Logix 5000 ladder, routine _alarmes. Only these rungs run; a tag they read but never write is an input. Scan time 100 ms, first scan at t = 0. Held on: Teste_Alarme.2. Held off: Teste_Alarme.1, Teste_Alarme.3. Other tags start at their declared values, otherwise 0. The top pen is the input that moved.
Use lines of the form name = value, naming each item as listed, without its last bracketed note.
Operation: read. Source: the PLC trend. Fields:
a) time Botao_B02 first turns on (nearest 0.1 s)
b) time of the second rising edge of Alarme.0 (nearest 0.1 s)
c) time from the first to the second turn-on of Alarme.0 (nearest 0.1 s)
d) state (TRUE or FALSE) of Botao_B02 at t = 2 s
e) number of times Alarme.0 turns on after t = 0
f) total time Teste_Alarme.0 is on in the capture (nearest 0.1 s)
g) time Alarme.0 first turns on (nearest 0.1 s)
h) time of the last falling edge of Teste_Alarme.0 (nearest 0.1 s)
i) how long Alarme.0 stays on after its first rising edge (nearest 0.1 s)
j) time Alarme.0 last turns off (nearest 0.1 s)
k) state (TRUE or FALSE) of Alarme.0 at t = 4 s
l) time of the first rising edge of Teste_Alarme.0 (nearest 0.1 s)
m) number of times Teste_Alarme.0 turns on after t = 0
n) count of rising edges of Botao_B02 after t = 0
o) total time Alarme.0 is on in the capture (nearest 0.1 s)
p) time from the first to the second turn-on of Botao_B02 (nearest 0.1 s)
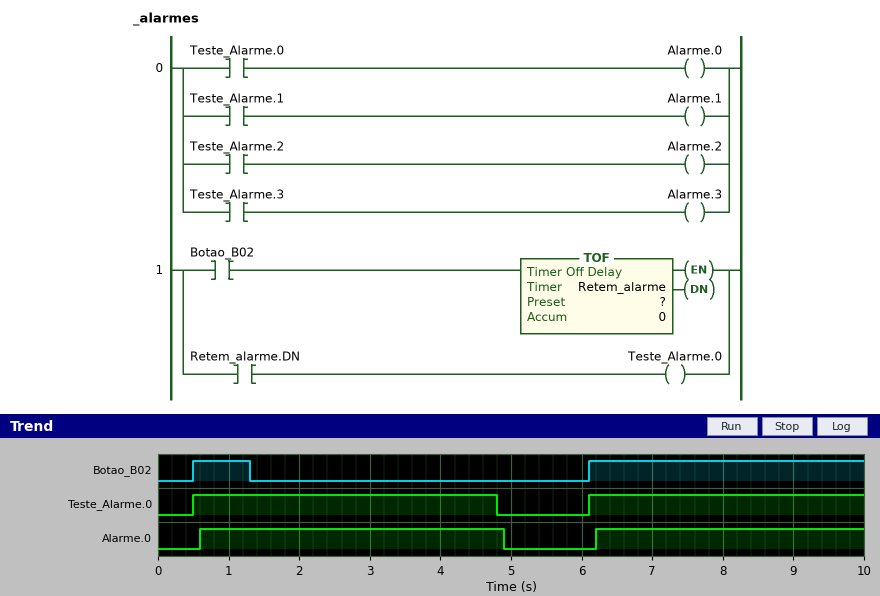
time Botao_B02 first turns on = 0.5 s
time of the second rising edge of Alarme.0 = 6.2 s
time from the first to the second turn-on of Alarme.0 = 5.6 s
state (TRUE or FALSE) of Botao_B02 at t = 2 s = FALSE
number of times Alarme.0 turns on after t = 0 = 2
total time Teste_Alarme.0 is on in the capture = 8.2 s
time Alarme.0 first turns on = 0.6 s
time of the last falling edge of Teste_Alarme.0 = 4.8 s
how long Alarme.0 stays on after its first rising edge = 4.3 s
time Alarme.0 last turns off = 4.9 s
state (TRUE or FALSE) of Alarme.0 at t = 4 s = TRUE
time of the first rising edge of Teste_Alarme.0 = 0.5 s
number of times Teste_Alarme.0 turns on after t = 0 = 2
count of rising edges of Botao_B02 after t = 0 = 2
total time Alarme.0 is on in the capture = 8.1 s
time from the first to the second turn-on of Botao_B02 = 5.6 s
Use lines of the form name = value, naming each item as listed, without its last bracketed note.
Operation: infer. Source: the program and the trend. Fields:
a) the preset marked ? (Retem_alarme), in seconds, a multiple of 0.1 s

the preset marked ? (Retem_alarme), in seconds, a multiple of 0.1 s = 3.5 s
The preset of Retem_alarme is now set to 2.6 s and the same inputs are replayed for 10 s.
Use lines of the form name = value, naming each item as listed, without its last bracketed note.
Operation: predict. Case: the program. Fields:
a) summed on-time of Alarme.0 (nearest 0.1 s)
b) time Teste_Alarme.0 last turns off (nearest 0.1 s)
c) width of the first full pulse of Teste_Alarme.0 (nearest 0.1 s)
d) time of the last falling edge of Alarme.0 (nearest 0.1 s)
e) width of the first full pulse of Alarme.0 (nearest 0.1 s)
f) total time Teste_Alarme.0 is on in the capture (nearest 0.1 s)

summed on-time of Alarme.0 = 7.2 s
time Teste_Alarme.0 last turns off = 3.9 s
width of the first full pulse of Teste_Alarme.0 = 3.4 s
time of the last falling edge of Alarme.0 = 4.0 s
width of the first full pulse of Alarme.0 = 3.4 s
total time Teste_Alarme.0 is on in the capture = 7.3 s
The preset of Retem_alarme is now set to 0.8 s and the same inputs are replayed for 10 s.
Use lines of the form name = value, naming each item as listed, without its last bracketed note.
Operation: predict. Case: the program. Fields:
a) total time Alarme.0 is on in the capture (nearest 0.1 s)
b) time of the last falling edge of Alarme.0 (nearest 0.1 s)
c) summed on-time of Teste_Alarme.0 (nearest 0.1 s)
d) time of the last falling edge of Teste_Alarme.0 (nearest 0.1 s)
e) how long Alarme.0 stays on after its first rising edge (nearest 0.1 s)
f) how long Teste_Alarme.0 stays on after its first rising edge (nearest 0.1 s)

total time Alarme.0 is on in the capture = 5.4 s
time of the last falling edge of Alarme.0 = 2.2 s
summed on-time of Teste_Alarme.0 = 5.5 s
time of the last falling edge of Teste_Alarme.0 = 2.1 s
how long Alarme.0 stays on after its first rising edge = 1.6 s
how long Teste_Alarme.0 stays on after its first rising edge = 1.6 s
